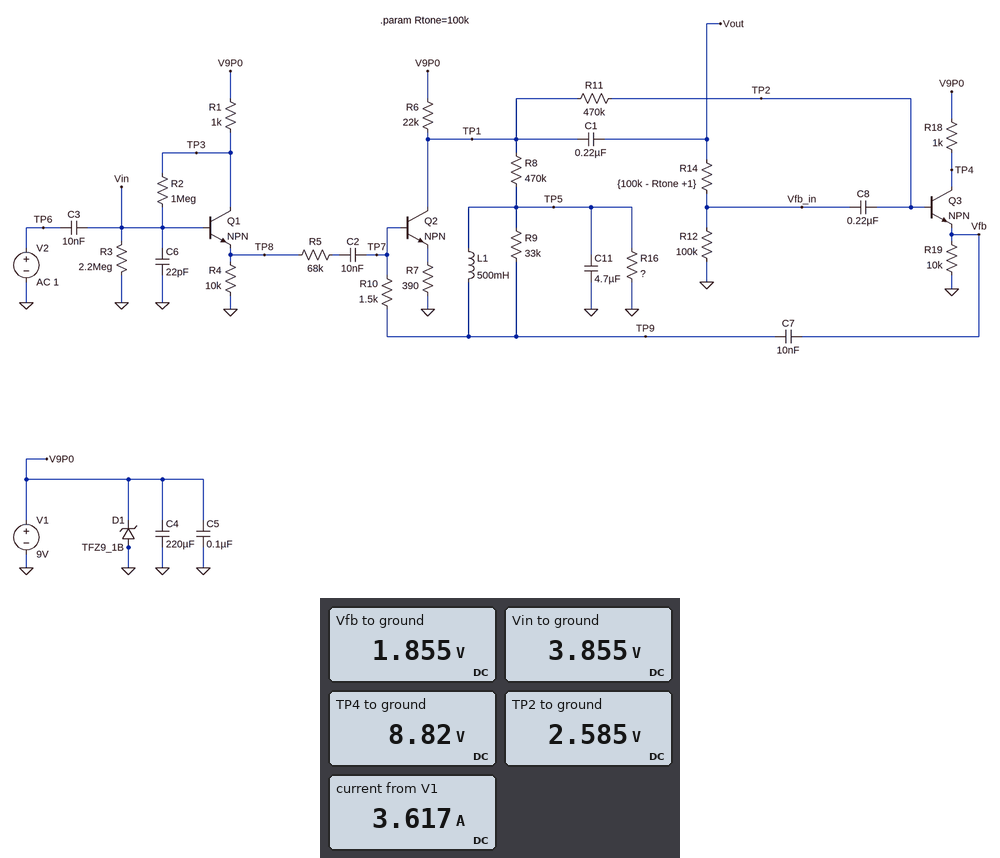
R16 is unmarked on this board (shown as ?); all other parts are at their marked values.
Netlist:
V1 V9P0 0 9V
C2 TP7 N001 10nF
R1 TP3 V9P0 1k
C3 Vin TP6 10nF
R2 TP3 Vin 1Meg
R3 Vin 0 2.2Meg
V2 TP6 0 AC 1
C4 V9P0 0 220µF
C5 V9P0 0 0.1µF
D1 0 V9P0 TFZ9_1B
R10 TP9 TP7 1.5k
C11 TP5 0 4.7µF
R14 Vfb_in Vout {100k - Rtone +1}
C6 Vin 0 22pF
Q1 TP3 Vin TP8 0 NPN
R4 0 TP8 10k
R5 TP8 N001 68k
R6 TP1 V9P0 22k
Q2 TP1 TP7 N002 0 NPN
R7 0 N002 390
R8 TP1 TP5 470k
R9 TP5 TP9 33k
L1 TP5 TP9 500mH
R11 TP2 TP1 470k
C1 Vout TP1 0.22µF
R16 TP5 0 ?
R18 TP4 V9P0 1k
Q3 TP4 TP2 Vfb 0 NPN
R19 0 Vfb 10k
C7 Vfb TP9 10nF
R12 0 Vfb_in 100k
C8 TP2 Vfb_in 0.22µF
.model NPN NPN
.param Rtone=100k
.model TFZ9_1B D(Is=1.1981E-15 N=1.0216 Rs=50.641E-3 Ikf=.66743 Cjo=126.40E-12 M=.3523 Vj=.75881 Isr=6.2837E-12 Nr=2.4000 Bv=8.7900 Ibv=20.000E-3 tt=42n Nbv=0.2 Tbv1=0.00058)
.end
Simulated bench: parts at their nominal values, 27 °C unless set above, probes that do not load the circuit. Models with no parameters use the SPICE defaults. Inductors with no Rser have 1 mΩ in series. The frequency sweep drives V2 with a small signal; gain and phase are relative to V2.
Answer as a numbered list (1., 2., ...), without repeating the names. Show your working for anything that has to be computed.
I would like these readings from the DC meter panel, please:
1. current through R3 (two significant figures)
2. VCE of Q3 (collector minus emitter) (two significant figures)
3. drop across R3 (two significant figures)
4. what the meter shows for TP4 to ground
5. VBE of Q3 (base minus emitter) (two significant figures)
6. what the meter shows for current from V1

1. (3.855 V) / 2.2 MΩ = 1.8 µA
2. 8.82 V - 1.855 V = 7.0 V
3. 3.855 V = 3.9 V
4. 8.82 V
5. 2.585 V - 1.855 V = 730 mV
6. 3.617 A
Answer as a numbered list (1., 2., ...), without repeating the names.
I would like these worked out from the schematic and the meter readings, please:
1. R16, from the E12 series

1. 270 kΩ
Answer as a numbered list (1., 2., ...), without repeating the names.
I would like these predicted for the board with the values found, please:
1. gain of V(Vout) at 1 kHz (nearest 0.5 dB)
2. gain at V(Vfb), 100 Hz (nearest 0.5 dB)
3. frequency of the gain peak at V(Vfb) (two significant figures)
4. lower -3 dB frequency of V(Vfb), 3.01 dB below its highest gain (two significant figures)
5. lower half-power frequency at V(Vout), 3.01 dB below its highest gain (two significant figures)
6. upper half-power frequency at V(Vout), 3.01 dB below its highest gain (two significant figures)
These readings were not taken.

1. -10.5 dB
2. -12.0 dB
3. 400 Hz
4. 390 Hz
5. 390 Hz
6. 420 Hz
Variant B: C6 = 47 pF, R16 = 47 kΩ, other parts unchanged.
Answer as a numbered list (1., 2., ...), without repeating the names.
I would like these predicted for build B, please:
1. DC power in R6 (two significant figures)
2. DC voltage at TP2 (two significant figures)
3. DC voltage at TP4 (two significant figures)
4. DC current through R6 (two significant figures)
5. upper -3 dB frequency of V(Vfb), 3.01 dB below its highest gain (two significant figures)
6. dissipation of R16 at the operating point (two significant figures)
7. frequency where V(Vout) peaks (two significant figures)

1. 61 µW
2. 5.6 V
3. 8.5 V
4. 53 µA
5. 620 Hz
6. 10 µW
7. 590 Hz
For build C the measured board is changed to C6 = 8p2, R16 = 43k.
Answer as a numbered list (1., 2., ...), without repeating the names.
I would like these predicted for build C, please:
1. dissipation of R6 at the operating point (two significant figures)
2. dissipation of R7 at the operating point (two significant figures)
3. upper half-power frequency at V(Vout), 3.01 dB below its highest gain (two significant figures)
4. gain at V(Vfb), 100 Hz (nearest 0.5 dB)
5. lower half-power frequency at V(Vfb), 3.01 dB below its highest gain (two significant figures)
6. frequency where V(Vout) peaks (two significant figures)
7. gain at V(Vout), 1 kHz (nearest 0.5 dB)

1. 32 µW
2. 120 nW
3. 760 Hz
4. -23.0 dB
5. 680 Hz
6. 720 Hz
7. -6.5 dB
